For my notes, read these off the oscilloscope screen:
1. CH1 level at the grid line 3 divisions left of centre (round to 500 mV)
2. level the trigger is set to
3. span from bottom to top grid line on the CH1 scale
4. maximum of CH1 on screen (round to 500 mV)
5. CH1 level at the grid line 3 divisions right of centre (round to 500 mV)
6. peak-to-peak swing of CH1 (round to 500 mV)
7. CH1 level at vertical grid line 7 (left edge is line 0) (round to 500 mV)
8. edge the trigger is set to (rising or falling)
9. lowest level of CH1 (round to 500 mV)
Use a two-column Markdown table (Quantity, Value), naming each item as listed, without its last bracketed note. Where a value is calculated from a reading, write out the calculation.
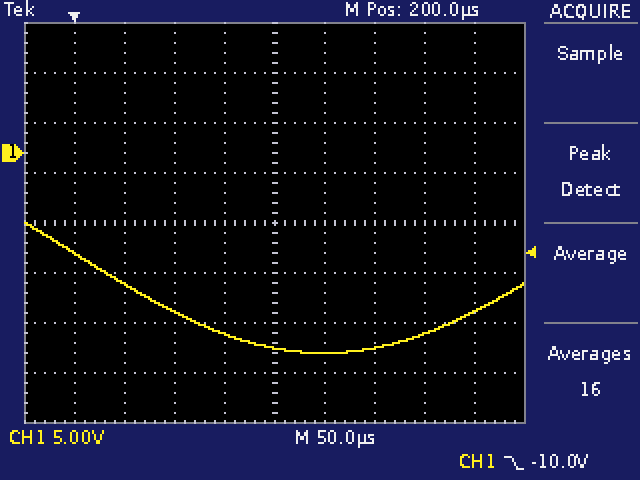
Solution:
| Quantity | Value |
|---|---|
| CH1 level at the grid line 3 divisions left of centre | -13.0 V |
| level the trigger is set to | -10.0 V |
| span from bottom to top grid line on the CH1 scale | 40 V |
| maximum of CH1 on screen | -7.0 V |
| CH1 level at the grid line 3 divisions right of centre | -18.0 V |
| peak-to-peak swing of CH1 | -7.0 V − (-20.0 V) = 13.0 V |
| CH1 level at vertical grid line 7 (left edge is line 0) | -19.5 V |
| edge the trigger is set to | falling |
| lowest level of CH1 | -20.0 V |
